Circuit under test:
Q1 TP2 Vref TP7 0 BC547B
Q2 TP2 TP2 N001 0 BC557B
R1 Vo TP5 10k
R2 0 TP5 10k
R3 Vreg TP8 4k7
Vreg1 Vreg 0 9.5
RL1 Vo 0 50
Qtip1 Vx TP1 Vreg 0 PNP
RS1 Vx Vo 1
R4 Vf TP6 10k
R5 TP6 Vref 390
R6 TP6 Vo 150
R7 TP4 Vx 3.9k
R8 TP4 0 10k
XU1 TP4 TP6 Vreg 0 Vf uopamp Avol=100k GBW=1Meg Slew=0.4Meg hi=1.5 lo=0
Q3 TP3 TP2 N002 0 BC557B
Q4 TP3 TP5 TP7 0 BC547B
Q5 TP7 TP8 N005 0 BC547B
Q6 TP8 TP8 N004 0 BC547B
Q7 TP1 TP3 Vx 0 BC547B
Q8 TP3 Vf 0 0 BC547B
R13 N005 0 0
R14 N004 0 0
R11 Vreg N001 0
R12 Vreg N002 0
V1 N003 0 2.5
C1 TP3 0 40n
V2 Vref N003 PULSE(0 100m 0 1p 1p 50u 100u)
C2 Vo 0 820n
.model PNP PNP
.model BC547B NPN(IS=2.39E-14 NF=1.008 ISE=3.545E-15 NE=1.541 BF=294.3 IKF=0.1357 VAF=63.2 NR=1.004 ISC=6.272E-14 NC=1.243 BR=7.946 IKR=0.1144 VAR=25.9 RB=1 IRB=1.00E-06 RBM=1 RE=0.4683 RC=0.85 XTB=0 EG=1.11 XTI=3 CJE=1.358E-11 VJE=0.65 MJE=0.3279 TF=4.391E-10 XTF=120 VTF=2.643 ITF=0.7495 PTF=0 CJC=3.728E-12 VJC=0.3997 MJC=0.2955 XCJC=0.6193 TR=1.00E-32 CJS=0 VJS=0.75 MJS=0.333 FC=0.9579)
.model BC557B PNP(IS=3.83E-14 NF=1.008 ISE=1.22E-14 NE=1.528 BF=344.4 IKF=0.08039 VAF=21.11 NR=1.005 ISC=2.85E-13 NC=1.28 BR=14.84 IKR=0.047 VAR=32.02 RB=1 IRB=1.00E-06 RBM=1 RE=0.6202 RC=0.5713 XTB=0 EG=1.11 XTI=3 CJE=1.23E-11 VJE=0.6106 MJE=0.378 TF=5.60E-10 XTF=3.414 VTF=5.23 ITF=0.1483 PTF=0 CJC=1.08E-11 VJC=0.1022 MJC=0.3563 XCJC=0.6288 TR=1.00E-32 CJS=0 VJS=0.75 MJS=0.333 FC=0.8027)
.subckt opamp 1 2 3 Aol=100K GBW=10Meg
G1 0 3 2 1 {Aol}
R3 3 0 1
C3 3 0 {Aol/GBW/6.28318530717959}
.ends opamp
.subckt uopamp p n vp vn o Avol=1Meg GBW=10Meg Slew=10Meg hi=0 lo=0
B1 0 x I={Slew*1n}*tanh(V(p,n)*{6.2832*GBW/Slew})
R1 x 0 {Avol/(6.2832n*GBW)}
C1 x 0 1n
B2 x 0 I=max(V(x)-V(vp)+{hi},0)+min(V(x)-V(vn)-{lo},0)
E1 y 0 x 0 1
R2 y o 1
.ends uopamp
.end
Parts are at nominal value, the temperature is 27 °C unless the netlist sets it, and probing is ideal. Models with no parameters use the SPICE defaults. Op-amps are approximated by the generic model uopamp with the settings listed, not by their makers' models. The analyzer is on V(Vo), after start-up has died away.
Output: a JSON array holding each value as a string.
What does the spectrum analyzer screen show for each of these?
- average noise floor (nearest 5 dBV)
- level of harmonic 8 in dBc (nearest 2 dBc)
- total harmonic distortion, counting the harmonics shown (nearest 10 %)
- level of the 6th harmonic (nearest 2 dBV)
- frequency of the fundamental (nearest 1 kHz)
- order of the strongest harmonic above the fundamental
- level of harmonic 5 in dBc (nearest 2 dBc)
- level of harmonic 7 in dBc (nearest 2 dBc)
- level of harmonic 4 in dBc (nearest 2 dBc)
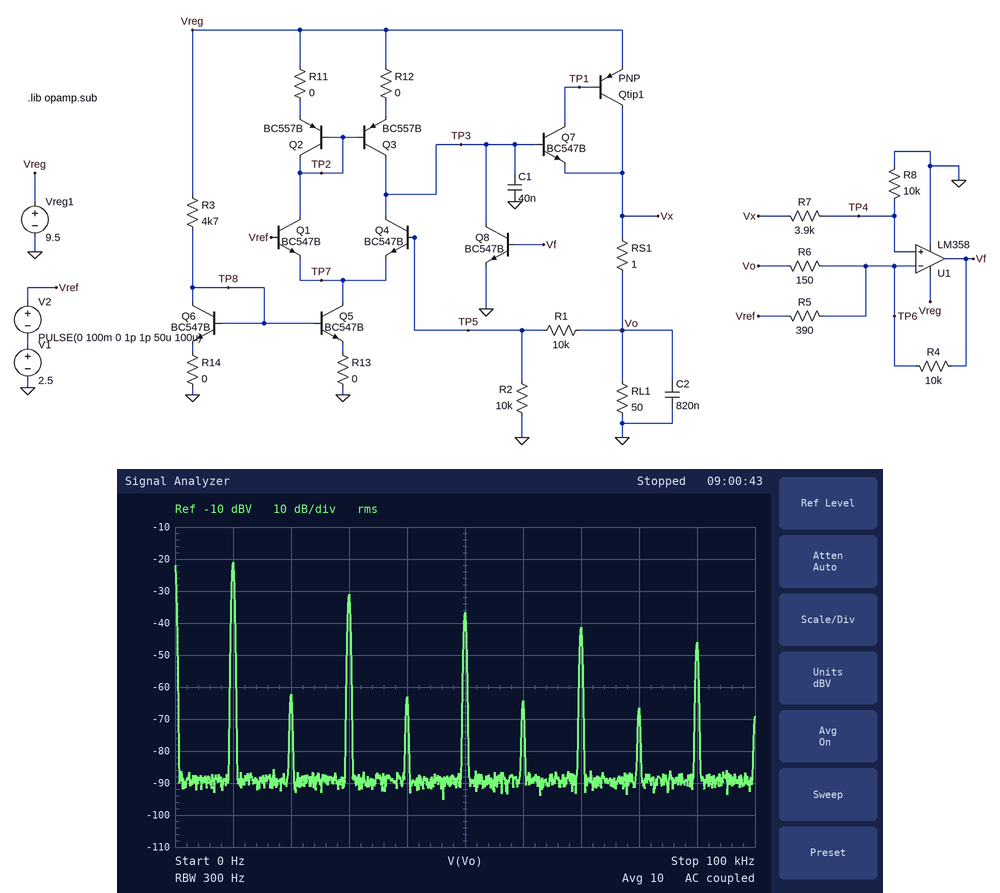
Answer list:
["-90 dBV", "-46 dBc", "40 %", "-64 dBV", "10 kHz", "3", "-16 dBc", "-20 dBc", "-42 dBc"]
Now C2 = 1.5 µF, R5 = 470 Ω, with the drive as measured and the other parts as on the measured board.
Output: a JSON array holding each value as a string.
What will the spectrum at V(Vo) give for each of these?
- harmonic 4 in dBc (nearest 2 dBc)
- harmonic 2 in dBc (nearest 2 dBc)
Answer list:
["-38 dBc", "-40 dBc"]
